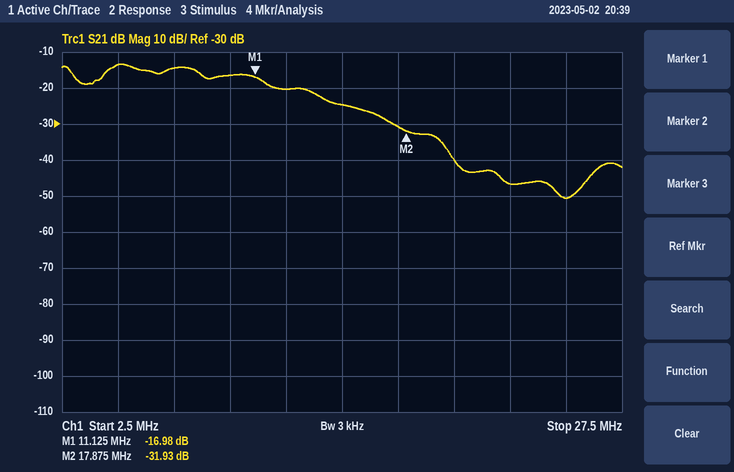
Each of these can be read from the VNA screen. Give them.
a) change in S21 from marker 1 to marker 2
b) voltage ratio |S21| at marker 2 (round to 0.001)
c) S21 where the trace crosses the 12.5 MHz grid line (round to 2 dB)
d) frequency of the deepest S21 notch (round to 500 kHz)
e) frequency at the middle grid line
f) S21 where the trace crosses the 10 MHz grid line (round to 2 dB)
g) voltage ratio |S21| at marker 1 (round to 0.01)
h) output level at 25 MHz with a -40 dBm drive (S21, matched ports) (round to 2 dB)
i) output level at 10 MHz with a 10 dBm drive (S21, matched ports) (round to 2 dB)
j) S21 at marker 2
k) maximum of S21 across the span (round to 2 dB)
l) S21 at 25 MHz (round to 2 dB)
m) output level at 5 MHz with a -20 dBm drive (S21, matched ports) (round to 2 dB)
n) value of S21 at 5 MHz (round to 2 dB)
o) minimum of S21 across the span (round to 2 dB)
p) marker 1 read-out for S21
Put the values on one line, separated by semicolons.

-14.95 dB; 0.025; -20 dB; 25.0 MHz; 15 MHz; -16 dB; 0.14; -90 dBm; -6 dBm; -31.93 dB; -14 dB; -50 dB; -34 dBm; -14 dB; -50 dB; -16.98 dB
